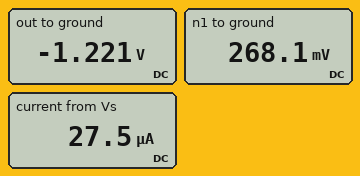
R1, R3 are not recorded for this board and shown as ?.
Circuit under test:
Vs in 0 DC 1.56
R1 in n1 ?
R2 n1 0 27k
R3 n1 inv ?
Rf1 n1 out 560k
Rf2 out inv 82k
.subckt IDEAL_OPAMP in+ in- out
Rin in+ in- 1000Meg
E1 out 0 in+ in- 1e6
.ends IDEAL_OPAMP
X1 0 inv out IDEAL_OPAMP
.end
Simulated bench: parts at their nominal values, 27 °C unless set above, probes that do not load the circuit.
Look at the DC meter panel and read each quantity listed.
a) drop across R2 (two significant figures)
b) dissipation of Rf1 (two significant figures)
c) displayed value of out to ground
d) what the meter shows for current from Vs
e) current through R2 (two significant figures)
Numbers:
270 mV
4.0 µW
-1.221 V
27.5 µA
9.9 µA
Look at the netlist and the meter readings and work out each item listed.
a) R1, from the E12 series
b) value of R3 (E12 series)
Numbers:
47 kΩ
18 kΩ
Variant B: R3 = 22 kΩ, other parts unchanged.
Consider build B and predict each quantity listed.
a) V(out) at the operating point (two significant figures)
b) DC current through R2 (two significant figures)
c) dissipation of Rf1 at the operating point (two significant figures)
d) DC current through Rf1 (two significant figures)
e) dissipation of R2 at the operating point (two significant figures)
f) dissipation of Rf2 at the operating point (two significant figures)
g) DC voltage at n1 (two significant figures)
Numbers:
-1.1 V
11 µA
3.5 µW
2.5 µA
3.2 µW
15 µW
300 mV
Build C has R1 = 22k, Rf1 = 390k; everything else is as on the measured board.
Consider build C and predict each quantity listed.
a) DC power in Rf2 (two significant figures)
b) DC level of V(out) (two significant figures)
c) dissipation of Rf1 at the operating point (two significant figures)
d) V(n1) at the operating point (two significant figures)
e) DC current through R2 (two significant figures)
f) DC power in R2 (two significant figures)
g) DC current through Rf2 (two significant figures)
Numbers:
55 µW
-2.1 V
17 µW
470 mV
17 µA
8.0 µW
26 µA
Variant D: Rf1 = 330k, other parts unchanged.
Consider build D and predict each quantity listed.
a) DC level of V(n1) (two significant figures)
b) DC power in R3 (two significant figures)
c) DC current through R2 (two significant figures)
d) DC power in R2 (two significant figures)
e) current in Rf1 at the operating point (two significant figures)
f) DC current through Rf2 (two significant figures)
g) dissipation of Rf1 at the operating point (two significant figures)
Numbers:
250 mV
3.6 µW
9.4 µA
2.4 µW
4.3 µA
14 µA
6.0 µW
